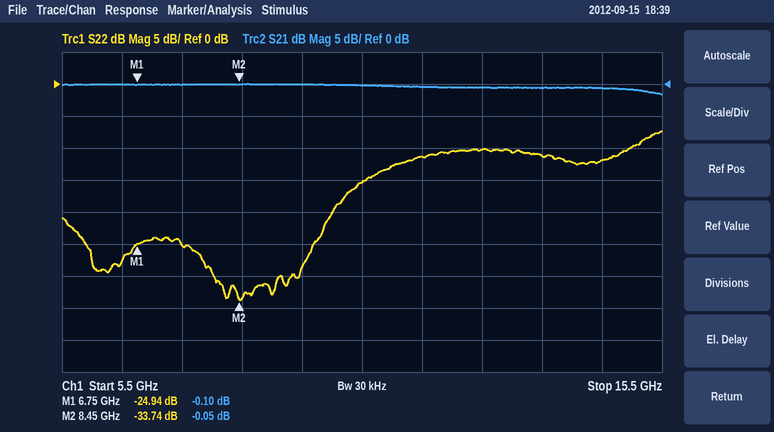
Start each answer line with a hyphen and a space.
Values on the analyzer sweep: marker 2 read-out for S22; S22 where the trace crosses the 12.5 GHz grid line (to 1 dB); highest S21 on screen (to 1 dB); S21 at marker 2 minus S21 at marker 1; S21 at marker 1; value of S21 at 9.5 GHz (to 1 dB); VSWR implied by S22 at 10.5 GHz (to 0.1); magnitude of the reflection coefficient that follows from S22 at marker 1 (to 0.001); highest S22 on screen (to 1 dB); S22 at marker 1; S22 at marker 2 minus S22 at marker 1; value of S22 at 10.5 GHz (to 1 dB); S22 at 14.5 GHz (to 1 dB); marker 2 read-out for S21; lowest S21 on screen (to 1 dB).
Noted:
- -33.74 dB
- -10 dB
- 0 dB
- 0.05 dB
- -0.10 dB
- 0 dB
- 1.4
- 0.057
- -7 dB
- -24.94 dB
- -8.80 dB
- -15 dB
- -12 dB
- -0.05 dB
- -2 dB
